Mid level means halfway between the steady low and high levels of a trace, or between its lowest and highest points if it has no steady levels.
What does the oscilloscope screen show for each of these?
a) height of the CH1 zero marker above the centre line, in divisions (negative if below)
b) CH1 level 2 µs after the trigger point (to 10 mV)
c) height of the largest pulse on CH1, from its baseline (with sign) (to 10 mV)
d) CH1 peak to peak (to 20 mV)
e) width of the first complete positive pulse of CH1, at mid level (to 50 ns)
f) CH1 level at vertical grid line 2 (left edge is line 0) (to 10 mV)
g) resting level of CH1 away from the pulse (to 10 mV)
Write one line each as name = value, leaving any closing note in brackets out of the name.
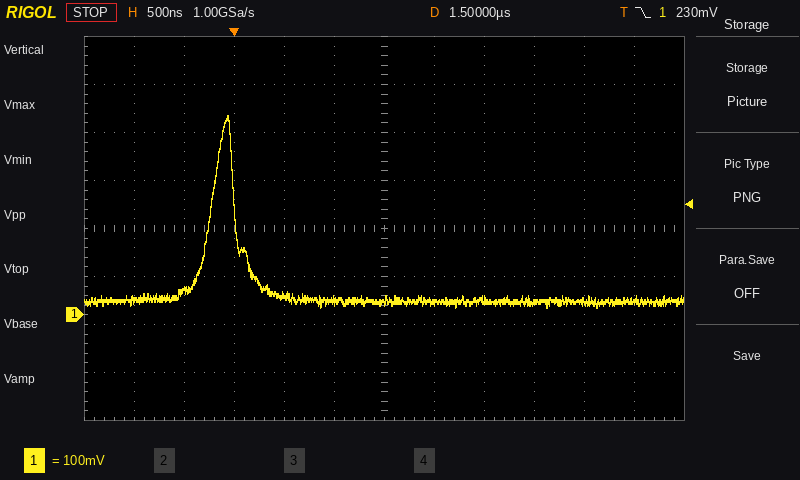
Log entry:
height of the CH1 zero marker above the centre line, in divisions = -1.8 div
CH1 level 2 µs after the trigger point = 30 mV
height of the largest pulse on CH1, from its baseline (with sign) = +390 mV
CH1 peak to peak = 400 mV
width of the first complete positive pulse of CH1, at mid level = 250 ns
CH1 level at vertical grid line 2 (left edge is line 0) = 50 mV
resting level of CH1 away from the pulse = 30 mV
